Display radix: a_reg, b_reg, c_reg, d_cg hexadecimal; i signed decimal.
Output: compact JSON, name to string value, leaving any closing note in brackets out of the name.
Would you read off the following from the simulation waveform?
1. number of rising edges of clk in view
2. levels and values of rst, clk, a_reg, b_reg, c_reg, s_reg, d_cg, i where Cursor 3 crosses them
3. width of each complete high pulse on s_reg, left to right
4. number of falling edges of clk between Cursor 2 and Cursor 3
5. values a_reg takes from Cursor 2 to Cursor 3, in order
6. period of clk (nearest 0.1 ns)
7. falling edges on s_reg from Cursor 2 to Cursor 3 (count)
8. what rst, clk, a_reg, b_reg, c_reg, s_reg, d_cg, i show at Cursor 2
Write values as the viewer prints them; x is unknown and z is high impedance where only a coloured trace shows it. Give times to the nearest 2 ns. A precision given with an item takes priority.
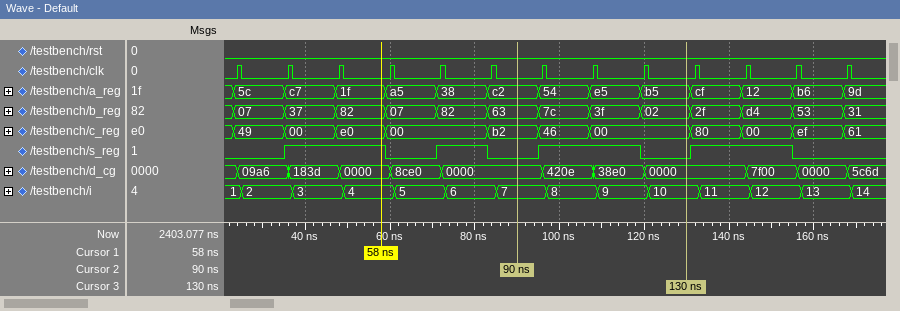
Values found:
{"number of rising edges of clk in view": "13", "levels and values of rst, clk, a_reg, b_reg, c_reg, s_reg, d_cg, i where Cursor 3 crosses them": "rst=0, clk=0, a_reg=b5, b_reg=02, c_reg=00, s_reg=0, d_cg=0000, i=10", "width of each complete high pulse on s_reg, left to right": "24 ns, 12 ns, 24 ns, 24 ns", "number of falling edges of clk between Cursor 2 and Cursor 3": "3", "values a_reg takes from Cursor 2 to Cursor 3, in order": "c2, 54, e5, b5", "period of clk": "12 ns", "falling edges on s_reg from Cursor 2 to Cursor 3": "1", "what rst, clk, a_reg, b_reg, c_reg, s_reg, d_cg, i show at Cursor 2": "rst=0, clk=0, a_reg=c2, b_reg=63, c_reg=b2, s_reg=0, d_cg=0000, i=7"}
